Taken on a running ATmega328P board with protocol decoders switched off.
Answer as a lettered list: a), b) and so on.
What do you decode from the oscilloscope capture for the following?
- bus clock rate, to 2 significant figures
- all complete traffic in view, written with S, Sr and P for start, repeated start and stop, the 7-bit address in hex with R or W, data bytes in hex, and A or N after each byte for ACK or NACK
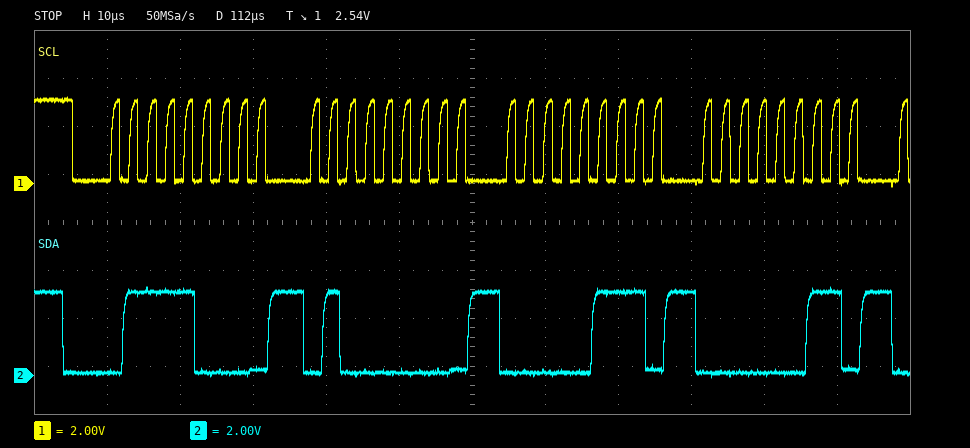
a) 400 kHz
b) S 3CW A 40 A 07 A 03 A
